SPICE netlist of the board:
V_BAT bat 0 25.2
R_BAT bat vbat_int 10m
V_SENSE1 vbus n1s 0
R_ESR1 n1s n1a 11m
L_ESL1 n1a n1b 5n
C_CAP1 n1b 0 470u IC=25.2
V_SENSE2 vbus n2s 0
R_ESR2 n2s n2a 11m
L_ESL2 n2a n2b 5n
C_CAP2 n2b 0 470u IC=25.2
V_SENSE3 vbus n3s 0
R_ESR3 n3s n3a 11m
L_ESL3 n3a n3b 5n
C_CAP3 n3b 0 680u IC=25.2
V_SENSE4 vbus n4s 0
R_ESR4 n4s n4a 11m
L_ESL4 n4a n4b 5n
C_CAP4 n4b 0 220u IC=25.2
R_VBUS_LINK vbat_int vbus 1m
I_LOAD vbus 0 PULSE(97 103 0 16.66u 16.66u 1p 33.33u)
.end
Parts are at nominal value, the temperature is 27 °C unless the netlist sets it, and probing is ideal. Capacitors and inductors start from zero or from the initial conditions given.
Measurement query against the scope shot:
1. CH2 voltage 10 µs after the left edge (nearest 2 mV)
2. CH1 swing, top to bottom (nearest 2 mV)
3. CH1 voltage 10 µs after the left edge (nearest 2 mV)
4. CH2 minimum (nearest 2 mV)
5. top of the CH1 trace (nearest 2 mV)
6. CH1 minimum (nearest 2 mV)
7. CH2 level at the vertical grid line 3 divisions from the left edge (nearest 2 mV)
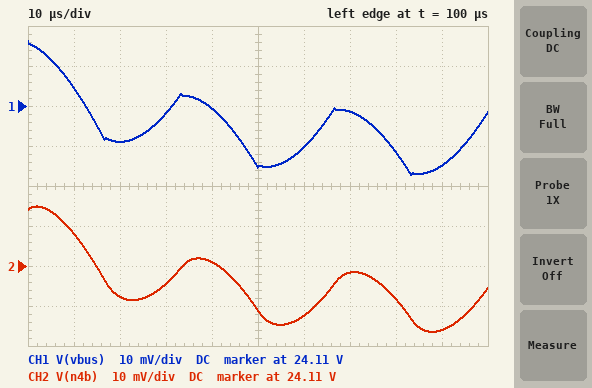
24.118 V
34 mV
24.114 V
24.094 V
24.126 V
24.092 V
24.106 V
